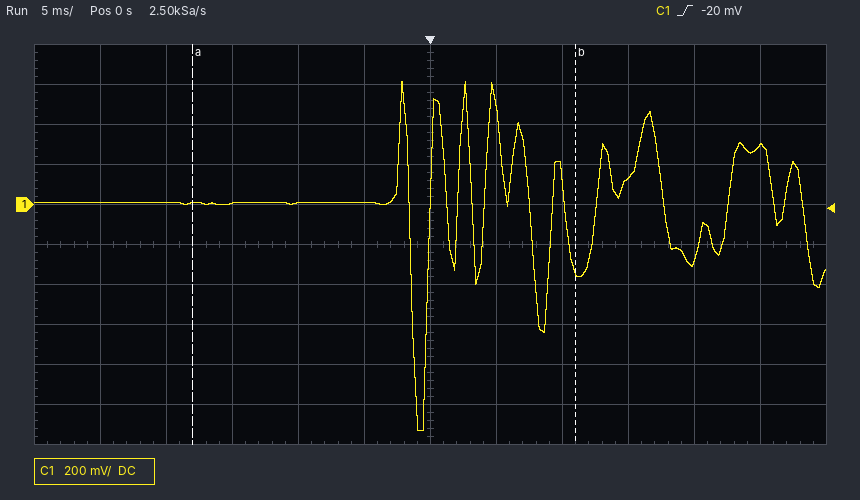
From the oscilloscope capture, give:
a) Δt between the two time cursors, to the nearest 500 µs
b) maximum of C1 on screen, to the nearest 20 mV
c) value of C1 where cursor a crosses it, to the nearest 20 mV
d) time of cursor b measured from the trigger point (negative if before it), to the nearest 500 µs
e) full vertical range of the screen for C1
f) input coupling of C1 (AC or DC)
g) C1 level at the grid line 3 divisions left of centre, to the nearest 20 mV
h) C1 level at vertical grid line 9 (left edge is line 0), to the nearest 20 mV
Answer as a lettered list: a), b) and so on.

a) 29.0 ms
b) 620 mV
c) 0 mV
d) +11.0 ms
e) 2 V
f) DC
g) 0 mV
h) 140 mV
